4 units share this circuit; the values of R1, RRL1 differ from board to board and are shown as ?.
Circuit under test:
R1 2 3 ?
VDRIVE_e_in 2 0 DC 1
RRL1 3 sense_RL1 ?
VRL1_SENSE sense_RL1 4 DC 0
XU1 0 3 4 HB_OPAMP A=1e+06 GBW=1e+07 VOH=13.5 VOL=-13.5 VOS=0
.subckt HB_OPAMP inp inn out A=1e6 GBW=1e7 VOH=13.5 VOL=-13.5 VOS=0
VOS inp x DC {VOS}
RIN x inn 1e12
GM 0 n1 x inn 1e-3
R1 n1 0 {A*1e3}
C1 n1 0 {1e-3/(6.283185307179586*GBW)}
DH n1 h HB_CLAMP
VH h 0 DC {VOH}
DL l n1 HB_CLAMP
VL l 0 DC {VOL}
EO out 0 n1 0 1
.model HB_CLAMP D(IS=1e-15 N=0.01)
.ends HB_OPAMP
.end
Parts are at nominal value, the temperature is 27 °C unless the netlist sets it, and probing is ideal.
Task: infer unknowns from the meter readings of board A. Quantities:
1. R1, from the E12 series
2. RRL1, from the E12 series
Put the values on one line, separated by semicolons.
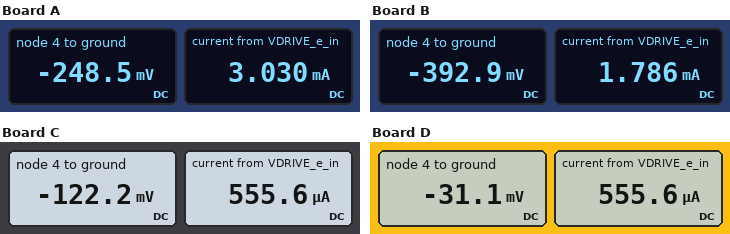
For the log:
330 Ω; 82 Ω
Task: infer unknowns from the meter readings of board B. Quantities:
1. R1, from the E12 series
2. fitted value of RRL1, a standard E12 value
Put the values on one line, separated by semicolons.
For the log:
560 Ω; 220 Ω
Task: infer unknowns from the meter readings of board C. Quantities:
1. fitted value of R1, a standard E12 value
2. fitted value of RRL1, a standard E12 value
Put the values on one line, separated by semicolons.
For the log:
1.8 kΩ; 220 Ω
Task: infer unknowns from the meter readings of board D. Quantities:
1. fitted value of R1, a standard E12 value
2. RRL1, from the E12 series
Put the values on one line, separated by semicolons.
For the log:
1.8 kΩ; 56 Ω
